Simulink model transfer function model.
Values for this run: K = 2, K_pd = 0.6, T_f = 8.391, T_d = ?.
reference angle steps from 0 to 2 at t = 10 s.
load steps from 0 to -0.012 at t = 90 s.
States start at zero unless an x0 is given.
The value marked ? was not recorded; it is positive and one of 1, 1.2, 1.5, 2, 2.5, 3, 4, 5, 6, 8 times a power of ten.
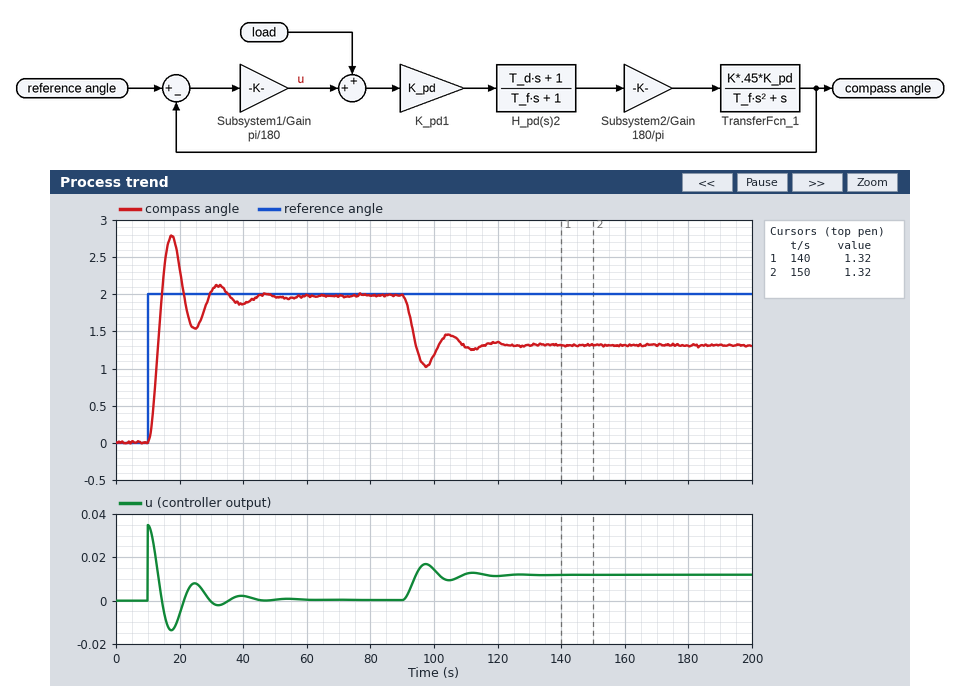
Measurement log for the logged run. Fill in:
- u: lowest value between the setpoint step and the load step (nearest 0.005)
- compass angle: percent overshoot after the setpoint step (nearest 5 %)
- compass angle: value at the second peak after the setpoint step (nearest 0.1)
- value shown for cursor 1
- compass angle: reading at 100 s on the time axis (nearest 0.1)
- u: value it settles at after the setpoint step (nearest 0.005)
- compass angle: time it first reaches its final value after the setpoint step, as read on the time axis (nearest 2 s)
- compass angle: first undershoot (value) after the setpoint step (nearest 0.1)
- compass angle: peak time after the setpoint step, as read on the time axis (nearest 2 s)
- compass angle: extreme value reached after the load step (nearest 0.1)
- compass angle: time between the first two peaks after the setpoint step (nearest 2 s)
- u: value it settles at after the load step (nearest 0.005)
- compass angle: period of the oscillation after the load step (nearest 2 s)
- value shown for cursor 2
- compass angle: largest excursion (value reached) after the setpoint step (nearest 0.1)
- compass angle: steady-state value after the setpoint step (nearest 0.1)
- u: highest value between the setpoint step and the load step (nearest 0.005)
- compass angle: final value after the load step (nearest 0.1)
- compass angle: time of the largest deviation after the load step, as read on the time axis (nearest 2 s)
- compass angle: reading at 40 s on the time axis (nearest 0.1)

-0.015
40 %
2.1
1.32
1.2
0.000
14 s
1.5
18 s
1.0
14 s
0.010
14 s
1.32
2.8
2.0
0.035
1.3
98 s
1.9
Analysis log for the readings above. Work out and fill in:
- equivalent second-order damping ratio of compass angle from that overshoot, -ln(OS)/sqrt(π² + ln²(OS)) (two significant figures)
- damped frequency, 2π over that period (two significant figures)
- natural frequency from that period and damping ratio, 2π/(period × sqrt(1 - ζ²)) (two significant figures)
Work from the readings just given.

0.28
0.45 rad/s
0.47 rad/s
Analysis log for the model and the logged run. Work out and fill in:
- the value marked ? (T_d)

40
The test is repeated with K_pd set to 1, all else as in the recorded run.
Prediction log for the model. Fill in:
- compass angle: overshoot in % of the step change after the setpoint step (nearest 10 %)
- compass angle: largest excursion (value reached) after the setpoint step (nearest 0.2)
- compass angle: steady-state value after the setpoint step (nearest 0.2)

60 %
3.2
2.0
